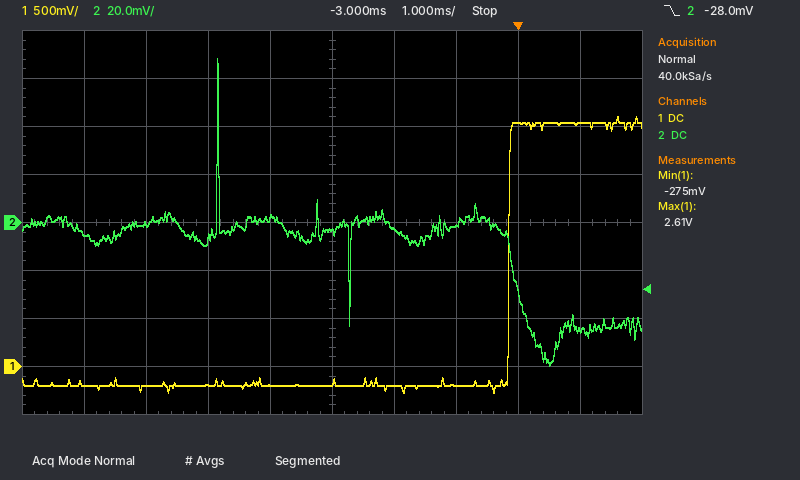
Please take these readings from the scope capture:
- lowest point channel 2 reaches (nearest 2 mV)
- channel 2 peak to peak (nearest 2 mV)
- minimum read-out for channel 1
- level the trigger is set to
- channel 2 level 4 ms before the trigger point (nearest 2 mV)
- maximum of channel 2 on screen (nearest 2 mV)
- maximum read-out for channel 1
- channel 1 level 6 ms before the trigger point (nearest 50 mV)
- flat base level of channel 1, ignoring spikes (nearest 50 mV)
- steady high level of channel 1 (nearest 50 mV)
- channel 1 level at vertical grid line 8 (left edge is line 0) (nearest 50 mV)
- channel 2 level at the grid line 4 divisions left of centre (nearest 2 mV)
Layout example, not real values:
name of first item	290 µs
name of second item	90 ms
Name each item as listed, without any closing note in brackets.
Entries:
lowest point channel 2 reaches	-60 mV
channel 2 peak to peak	128 mV
minimum read-out for channel 1	-275 mV
level the trigger is set to	-28.0 mV
channel 2 level 4 ms before the trigger point	2 mV
maximum of channel 2 on screen	68 mV
maximum read-out for channel 1	2.61 V
channel 1 level 6 ms before the trigger point	-200 mV
flat base level of channel 1, ignoring spikes	-200 mV
steady high level of channel 1	2.55 V
channel 1 level at vertical grid line 8 (left edge is line 0)	2.55 V
channel 2 level at the grid line 4 divisions left of centre	-4 mV
